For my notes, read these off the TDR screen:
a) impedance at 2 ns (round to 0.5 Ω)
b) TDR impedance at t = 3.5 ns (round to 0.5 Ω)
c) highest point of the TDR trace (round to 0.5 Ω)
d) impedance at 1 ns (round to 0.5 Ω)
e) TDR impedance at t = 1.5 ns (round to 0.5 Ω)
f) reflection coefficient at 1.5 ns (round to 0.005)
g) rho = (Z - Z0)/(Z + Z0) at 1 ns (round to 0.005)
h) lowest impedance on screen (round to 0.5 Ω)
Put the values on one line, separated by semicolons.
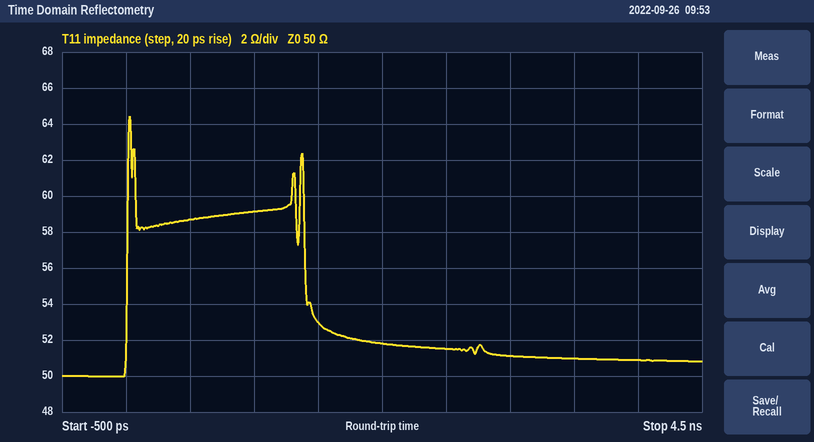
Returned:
52.0 Ω; 51.0 Ω; 64.5 Ω; 59.0 Ω; 53.0 Ω; +0.030; +0.085; 50.0 Ω
